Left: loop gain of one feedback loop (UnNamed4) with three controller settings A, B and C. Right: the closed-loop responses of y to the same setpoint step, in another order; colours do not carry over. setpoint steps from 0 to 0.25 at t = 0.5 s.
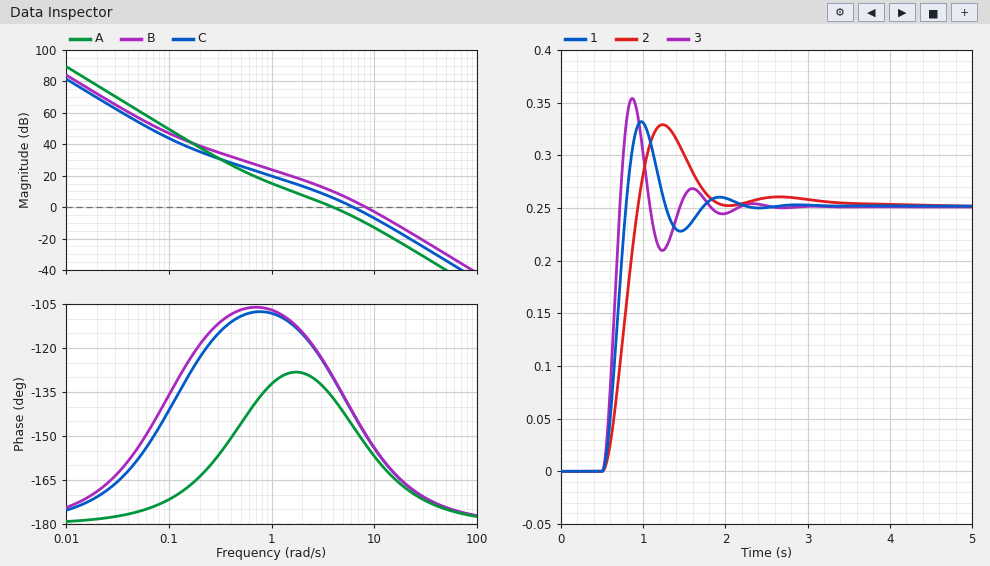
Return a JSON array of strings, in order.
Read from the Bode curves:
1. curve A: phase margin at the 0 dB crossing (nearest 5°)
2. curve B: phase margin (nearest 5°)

["45°", "30°"]
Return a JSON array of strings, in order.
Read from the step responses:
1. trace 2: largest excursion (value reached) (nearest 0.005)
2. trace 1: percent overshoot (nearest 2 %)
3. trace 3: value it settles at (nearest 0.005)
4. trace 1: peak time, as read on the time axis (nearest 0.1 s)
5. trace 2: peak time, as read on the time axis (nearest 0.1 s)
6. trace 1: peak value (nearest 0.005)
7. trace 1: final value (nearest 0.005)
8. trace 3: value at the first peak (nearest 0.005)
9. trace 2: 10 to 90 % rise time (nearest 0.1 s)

["0.330", "32 %", "0.250", "1.0 s", "1.2 s", "0.330", "0.250", "0.355", "0.3 s"]
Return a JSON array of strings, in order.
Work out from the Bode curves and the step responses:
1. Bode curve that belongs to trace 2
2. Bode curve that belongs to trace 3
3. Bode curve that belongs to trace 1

["A", "B", "C"]
